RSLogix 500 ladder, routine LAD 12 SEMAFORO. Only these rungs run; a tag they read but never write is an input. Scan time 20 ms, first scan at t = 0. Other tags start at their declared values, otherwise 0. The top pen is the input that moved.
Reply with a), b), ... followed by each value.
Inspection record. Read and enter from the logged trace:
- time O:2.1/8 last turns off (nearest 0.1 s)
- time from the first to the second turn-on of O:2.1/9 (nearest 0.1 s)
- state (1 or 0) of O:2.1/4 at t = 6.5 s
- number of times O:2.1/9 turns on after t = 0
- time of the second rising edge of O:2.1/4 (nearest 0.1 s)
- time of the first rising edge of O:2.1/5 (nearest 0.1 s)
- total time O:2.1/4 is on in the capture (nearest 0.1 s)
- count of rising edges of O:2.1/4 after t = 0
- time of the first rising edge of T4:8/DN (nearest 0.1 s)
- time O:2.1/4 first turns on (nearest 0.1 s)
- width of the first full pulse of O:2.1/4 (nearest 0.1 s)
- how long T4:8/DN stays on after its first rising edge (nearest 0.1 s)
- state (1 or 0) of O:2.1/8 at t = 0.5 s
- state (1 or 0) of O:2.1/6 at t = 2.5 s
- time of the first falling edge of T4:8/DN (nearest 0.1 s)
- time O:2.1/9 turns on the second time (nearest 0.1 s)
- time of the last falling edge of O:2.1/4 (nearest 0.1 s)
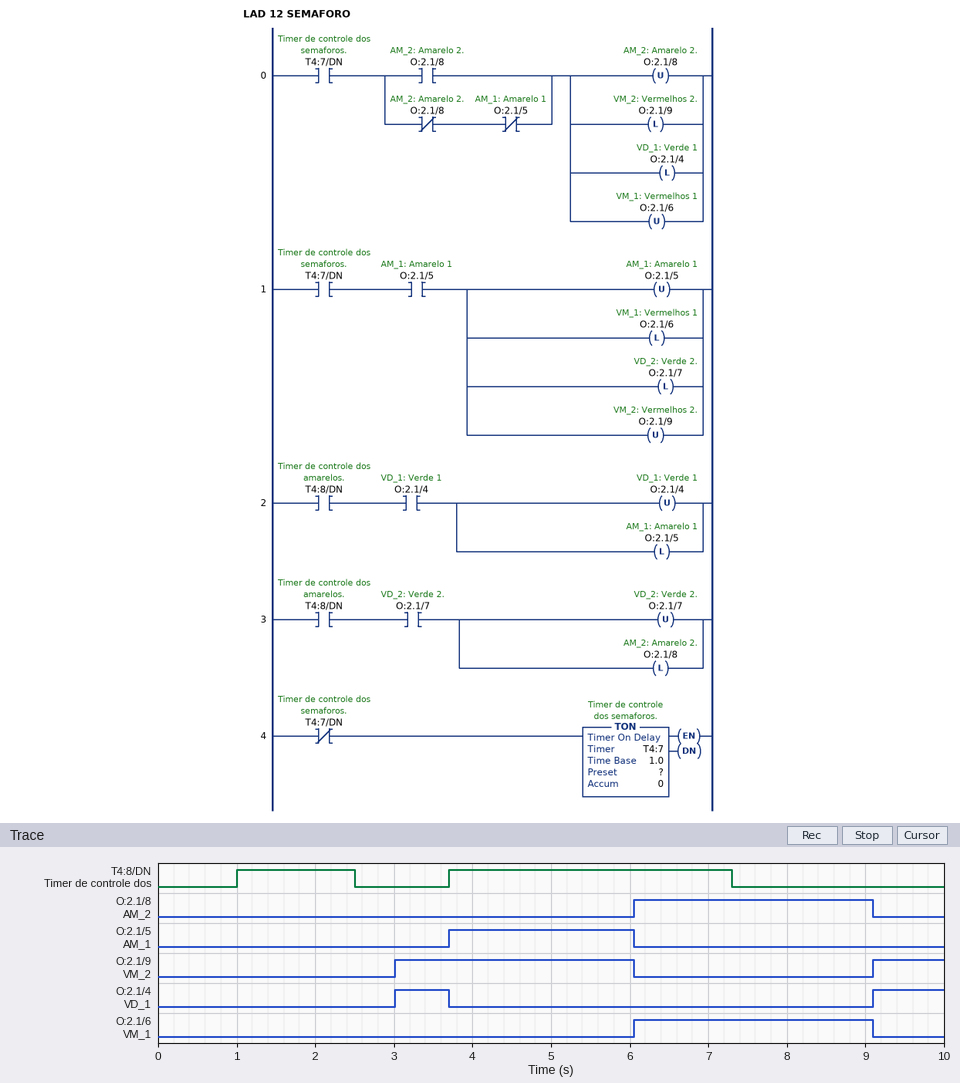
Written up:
a) 9.1 s
b) 6.1 s
c) 0
d) 2
e) 9.1 s
f) 3.7 s
g) 1.6 s
h) 2
i) 1.0 s
j) 3.0 s
k) 0.7 s
l) 1.5 s
m) 0
n) 0
o) 2.5 s
p) 9.1 s
q) 3.7 s
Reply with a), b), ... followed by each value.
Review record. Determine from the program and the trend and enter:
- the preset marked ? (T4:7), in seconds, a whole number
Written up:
a) 3 s
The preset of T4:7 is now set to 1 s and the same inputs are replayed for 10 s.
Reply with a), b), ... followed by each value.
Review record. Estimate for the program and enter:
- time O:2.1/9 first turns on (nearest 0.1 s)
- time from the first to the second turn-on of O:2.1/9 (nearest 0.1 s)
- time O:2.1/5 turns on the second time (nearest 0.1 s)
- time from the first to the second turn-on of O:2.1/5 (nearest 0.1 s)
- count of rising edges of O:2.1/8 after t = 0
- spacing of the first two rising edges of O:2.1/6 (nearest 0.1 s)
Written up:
a) 1.0 s
b) 2.1 s
c) 3.7 s
d) 2.7 s
e) 3
f) 2.1 s
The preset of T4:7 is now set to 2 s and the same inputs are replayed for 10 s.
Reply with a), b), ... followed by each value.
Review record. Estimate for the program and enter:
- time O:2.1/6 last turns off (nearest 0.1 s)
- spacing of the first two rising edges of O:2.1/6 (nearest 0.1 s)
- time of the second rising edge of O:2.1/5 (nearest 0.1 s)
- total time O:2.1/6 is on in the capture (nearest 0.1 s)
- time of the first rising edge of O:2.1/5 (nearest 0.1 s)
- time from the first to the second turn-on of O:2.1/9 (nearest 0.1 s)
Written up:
a) 6.1 s
b) 4.1 s
c) 6.1 s
d) 3.9 s
e) 2.0 s
f) 4.1 s
